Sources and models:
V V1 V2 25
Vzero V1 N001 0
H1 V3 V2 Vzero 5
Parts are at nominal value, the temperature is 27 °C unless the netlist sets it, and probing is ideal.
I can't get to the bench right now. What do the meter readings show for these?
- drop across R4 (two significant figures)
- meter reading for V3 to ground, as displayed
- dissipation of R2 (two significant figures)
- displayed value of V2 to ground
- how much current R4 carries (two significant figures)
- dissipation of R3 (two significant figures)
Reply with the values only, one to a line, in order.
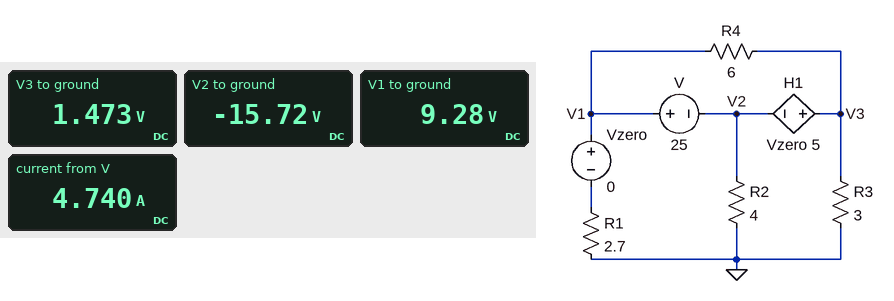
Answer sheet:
7.8 V
1.473 V
62 W
-15.72 V
1.3 A
720 mW
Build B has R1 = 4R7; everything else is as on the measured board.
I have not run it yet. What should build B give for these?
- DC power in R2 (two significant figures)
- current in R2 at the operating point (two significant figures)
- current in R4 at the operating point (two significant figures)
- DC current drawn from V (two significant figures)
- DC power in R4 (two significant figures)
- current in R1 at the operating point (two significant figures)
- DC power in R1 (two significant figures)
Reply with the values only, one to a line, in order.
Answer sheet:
38 W
3.1 A
1.9 A
4.6 A
22 W
2.7 A
34 W
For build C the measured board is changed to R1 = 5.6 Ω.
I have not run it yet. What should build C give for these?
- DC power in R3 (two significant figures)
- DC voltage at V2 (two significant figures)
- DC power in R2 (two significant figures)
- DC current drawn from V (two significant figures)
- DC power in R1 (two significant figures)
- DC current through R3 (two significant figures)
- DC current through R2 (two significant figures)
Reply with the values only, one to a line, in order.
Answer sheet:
370 mW
-11 V
32 W
4.6 A
34 W
350 mA
2.8 A
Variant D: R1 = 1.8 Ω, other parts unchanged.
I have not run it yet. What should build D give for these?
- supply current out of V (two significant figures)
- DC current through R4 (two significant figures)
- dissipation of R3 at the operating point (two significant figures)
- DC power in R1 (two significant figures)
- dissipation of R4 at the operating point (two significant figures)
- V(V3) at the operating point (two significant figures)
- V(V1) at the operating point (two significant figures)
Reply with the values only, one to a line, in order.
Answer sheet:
4.8 A
900 mA
940 mW
28 W
4.8 W
1.7 V
7.1 V
